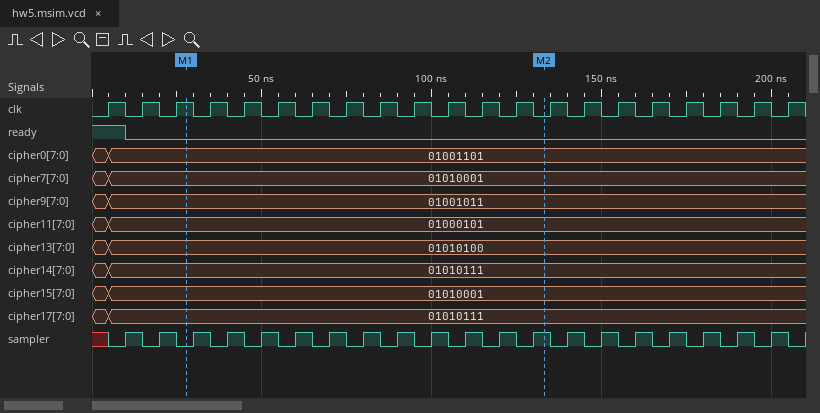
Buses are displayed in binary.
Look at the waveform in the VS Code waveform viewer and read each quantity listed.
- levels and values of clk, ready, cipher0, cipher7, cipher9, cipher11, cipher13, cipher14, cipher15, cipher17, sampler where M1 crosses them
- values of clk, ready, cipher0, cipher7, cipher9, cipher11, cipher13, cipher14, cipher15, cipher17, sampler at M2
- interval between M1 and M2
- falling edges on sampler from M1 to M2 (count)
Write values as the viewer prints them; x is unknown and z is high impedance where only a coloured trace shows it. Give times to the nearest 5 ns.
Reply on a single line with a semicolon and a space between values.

clk=1, ready=0, cipher0=01001101, cipher7=01010001, cipher9=01001011, cipher11=01000101, cipher13=01010100, cipher14=01010111, cipher15=01010001, cipher17=01010111, sampler=0; clk=0, ready=0, cipher0=01001101, cipher7=01010001, cipher9=01001011, cipher11=01000101, cipher13=01010100, cipher14=01010111, cipher15=01010001, cipher17=01010111, sampler=1; 105 ns; 10
